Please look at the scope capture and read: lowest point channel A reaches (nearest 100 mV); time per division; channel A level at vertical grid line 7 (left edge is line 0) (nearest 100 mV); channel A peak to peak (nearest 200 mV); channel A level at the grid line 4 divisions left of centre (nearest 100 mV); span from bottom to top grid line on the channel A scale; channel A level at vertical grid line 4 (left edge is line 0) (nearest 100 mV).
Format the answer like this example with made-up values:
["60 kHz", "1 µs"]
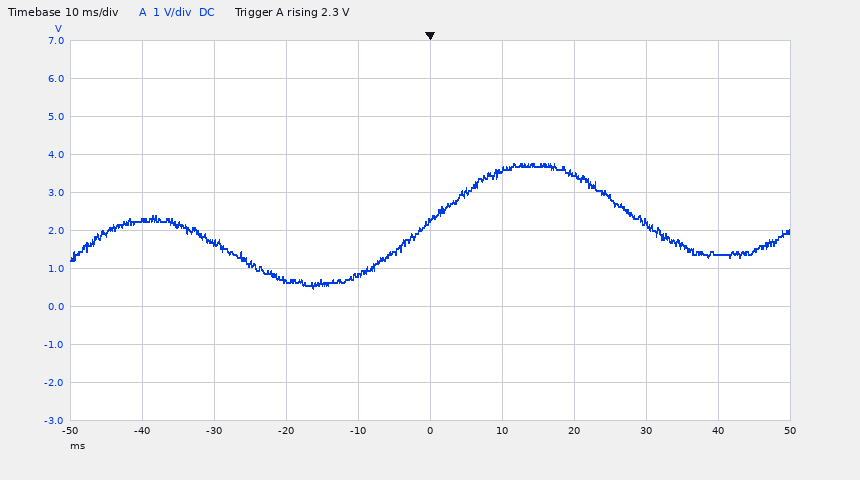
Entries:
["500 mV", "10 ms", "3.5 V", "3.2 V", "2.3 V", "10 V", "800 mV"]
